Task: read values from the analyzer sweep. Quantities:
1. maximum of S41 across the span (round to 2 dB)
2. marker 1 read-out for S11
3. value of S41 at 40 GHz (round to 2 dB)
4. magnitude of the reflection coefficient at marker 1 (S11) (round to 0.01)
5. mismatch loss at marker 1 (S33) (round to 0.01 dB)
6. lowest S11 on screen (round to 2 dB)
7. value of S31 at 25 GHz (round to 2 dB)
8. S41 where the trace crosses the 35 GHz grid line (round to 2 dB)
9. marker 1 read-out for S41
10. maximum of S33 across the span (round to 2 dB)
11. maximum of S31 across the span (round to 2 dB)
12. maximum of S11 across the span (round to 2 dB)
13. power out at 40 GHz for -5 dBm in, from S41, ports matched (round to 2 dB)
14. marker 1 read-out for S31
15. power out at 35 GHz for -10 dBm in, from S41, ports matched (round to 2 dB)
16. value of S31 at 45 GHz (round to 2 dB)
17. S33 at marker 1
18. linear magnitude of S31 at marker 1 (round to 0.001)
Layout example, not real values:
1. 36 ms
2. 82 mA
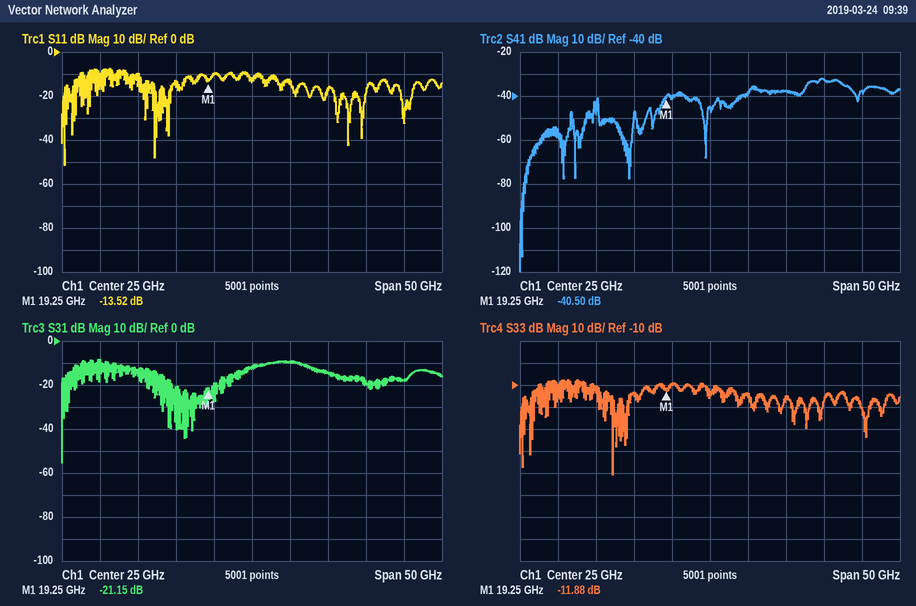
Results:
1. -32 dB
2. -13.52 dB
3. -32 dB
4. 0.21
5. 0.29 dB
6. -52 dB
7. -12 dB
8. -38 dB
9. -40.50 dB
10. -8 dB
11. -8 dB
12. -8 dB
13. -38 dBm
14. -21.15 dB
15. -48 dBm
16. -18 dB
17. -11.88 dB
18. 0.088
